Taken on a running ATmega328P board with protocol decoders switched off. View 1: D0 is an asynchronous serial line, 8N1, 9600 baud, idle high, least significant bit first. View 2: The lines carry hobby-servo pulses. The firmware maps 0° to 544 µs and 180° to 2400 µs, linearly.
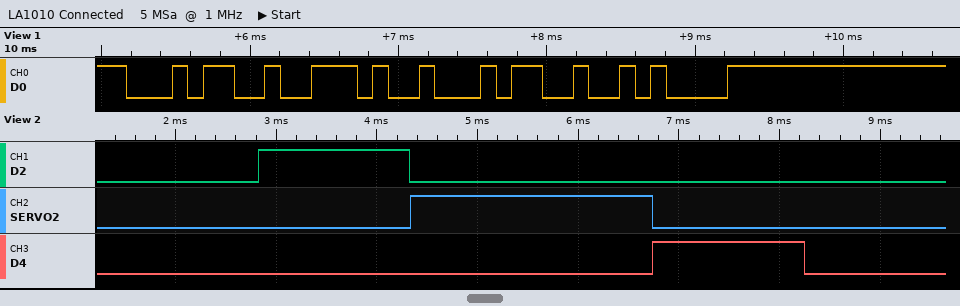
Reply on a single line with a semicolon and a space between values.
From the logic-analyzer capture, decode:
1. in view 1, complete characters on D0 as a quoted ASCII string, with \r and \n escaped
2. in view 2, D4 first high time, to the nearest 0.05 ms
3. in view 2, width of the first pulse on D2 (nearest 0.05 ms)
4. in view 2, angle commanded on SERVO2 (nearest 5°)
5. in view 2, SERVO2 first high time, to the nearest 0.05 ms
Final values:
"4.4\n"; 1.50 ms; 1.50 ms; 180°; 2.40 ms
